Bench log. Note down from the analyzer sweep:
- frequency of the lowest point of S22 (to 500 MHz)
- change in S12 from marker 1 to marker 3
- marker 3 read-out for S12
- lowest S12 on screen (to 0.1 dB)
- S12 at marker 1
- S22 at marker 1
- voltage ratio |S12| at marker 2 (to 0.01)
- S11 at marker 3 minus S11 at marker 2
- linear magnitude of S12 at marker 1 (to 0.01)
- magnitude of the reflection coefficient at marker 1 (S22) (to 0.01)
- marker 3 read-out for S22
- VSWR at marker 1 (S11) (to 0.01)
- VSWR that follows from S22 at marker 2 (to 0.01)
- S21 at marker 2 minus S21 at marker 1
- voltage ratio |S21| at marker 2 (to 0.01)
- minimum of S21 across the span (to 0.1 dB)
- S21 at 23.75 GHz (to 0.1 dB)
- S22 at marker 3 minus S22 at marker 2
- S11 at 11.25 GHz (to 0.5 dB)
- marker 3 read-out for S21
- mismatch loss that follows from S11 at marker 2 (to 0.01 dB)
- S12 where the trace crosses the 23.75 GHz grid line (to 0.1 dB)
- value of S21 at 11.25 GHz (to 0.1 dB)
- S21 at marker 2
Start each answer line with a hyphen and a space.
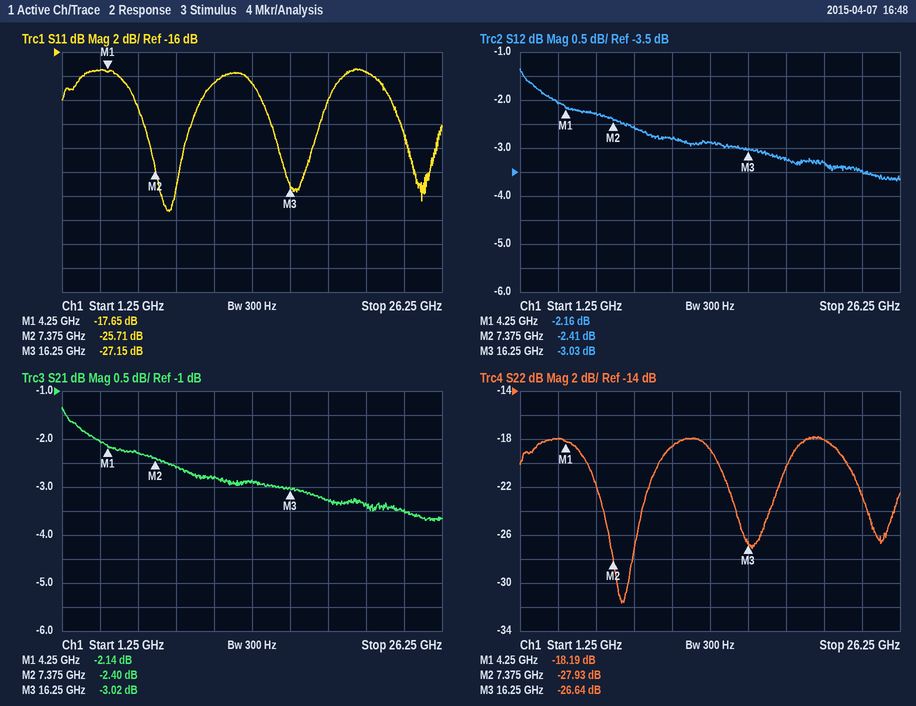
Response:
- 8.0 GHz
- -0.87 dB
- -3.03 dB
- -3.7 dB
- -2.16 dB
- -18.19 dB
- 0.76
- -1.44 dB
- 0.78
- 0.12
- -26.64 dB
- 1.30
- 1.08
- -0.26 dB
- 0.76
- -3.7 dB
- -3.5 dB
- 1.29 dB
- -18.5 dB
- -3.02 dB
- 0.01 dB
- -3.5 dB
- -2.8 dB
- -2.40 dB
